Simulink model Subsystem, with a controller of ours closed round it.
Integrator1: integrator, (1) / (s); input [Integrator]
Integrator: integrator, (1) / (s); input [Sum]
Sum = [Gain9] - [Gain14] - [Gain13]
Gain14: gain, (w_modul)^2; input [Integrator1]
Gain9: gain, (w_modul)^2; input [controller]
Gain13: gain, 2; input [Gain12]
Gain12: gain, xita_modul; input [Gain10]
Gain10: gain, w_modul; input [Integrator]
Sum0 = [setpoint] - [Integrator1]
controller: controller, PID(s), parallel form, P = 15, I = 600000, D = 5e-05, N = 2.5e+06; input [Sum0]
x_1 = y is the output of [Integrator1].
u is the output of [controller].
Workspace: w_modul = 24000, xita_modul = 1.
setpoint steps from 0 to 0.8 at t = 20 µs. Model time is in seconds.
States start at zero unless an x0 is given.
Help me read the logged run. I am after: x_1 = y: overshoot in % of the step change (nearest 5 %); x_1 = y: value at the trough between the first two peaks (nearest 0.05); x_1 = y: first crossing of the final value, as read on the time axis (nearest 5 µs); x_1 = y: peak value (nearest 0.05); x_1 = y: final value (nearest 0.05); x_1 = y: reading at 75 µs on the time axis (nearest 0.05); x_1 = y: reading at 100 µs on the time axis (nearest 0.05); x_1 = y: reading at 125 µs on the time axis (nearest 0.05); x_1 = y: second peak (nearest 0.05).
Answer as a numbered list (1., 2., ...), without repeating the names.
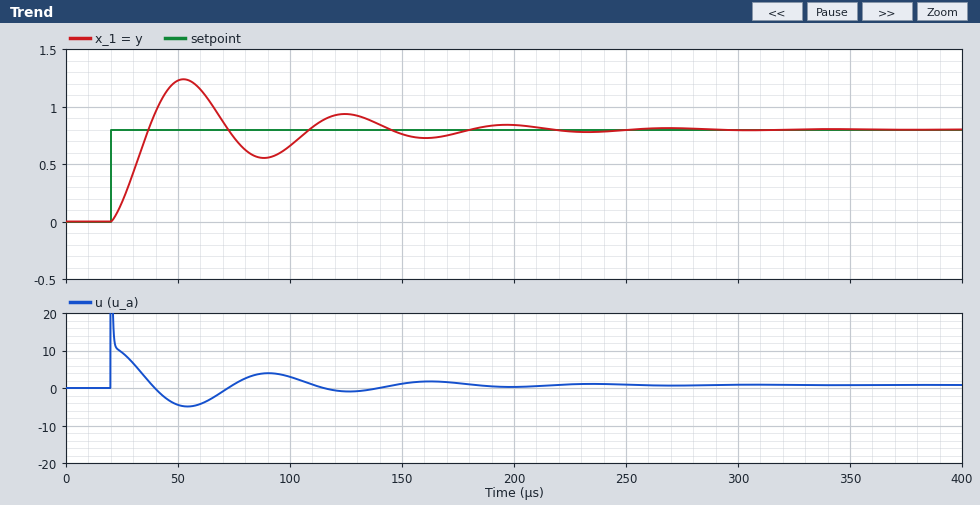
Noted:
1. 55 %
2. 0.55
3. 35 µs
4. 1.25
5. 0.80
6. 0.75
7. 0.65
8. 0.95
9. 0.95
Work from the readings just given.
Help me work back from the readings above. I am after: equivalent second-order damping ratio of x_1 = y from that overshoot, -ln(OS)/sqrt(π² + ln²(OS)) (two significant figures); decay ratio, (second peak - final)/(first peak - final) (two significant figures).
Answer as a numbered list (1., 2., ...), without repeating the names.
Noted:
1. 0.19
2. 0.33
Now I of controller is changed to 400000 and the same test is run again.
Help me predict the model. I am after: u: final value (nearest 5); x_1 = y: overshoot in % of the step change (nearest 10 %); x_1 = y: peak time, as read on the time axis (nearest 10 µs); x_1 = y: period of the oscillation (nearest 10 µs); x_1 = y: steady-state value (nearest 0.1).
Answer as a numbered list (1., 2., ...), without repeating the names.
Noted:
1. 0
2. 40 %
3. 50 µs
4. 70 µs
5. 0.8
